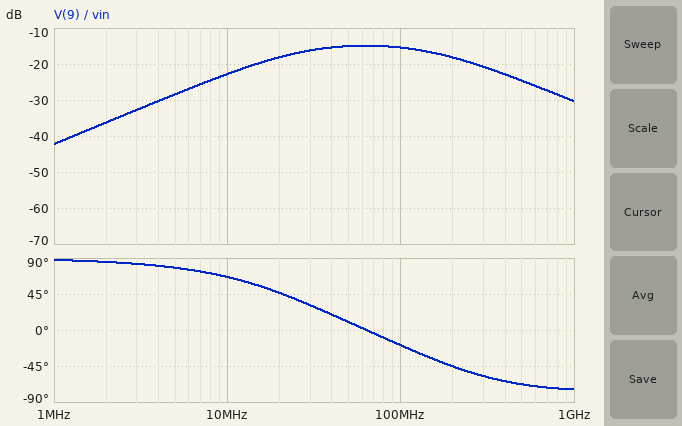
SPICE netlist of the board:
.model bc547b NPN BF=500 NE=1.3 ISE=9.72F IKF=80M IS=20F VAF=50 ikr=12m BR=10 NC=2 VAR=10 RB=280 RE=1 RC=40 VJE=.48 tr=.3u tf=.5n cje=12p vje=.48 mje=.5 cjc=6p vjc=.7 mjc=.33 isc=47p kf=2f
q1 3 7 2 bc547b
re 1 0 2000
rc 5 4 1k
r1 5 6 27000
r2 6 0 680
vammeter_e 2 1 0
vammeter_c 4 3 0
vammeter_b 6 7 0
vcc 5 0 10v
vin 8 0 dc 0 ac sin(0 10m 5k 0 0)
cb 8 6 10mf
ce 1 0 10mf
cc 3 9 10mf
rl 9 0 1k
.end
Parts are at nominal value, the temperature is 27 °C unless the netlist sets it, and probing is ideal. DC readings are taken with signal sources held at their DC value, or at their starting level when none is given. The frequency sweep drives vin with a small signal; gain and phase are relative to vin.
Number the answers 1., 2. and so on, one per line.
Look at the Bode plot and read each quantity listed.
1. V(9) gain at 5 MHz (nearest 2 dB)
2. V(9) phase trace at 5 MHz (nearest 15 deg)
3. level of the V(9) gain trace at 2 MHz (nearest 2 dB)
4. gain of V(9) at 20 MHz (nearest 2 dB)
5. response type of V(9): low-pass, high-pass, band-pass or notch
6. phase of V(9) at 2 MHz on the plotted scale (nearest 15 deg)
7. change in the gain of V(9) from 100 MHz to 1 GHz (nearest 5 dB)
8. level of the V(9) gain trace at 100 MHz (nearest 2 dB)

1. -28 dB
2. 75 deg
3. -36 dB
4. -18 dB
5. band-pass
6. 90 deg
7. -15 dB
8. -16 dB
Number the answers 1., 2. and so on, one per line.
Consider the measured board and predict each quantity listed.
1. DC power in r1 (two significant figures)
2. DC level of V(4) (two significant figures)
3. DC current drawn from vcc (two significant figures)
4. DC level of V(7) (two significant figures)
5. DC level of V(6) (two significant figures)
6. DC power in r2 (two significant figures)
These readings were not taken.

1. 3.5 mW
2. 10 V
3. 360 µA
4. 250 mV
5. 250 mV
6. 89 µW
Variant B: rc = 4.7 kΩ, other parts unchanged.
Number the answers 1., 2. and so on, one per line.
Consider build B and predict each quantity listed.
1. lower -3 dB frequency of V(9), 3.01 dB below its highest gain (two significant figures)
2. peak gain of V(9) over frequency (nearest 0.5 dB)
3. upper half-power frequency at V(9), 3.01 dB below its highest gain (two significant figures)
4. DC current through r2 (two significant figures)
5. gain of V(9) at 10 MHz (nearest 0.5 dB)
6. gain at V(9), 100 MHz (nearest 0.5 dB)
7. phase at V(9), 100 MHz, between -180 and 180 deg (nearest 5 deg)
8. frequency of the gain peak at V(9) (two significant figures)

1. 18 MHz
2. -11.5 dB
3. 140 MHz
4. 360 µA
5. -18.5 dB
6. -13.0 dB
7. -30 deg
8. 50 MHz
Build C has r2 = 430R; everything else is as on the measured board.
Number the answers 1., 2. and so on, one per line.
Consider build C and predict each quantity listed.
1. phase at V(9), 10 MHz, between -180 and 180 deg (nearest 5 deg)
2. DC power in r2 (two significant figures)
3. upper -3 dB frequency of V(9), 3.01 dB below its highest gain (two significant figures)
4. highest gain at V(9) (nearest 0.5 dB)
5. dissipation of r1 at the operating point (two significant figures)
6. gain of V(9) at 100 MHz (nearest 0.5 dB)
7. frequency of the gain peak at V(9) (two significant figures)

1. 70 deg
2. 57 µW
3. 200 MHz
4. -14.0 dB
5. 3.6 mW
6. -14.5 dB
7. 68 MHz
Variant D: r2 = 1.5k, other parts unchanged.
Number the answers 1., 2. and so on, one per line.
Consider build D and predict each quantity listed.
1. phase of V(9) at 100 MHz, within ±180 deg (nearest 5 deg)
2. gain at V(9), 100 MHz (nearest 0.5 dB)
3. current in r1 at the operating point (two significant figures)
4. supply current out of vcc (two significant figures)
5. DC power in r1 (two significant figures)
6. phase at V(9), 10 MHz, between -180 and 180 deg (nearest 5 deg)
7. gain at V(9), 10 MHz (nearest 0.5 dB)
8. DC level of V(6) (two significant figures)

1. -15 deg
2. -18.5 dB
3. 350 µA
4. 360 µA
5. 3.3 mW
6. 120 deg
7. -16.0 dB
8. 530 mV
